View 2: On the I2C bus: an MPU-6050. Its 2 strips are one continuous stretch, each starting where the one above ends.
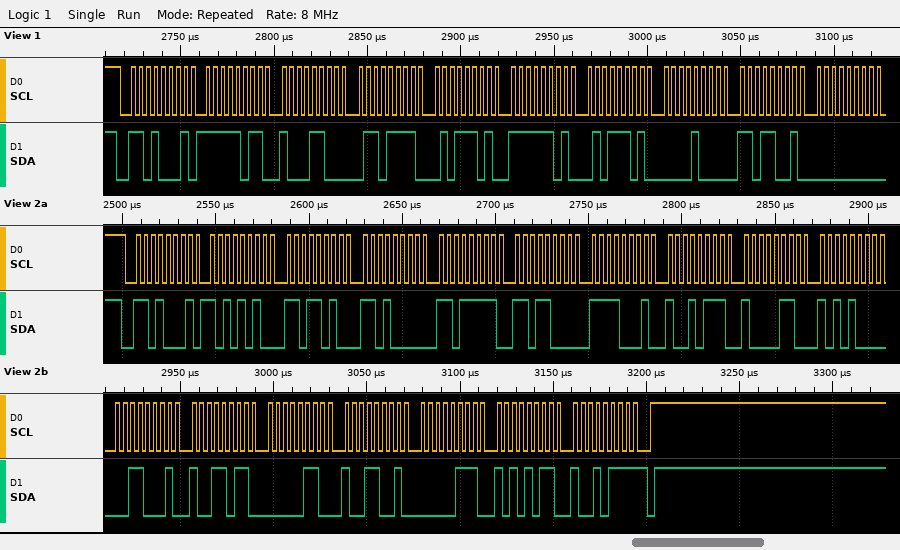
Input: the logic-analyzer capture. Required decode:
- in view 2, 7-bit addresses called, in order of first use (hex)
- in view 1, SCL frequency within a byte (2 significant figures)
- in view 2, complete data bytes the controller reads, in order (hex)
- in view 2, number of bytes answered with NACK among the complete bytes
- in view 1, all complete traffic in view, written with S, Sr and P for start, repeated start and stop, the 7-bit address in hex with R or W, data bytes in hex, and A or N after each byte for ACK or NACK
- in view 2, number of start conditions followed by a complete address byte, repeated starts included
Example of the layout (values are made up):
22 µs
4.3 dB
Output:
0x68
250 kHz
AA DA D0 DF D8 F1 97 86 A8 31 9B 06 99 07 AB 97
1
S 68R A FB A 8C A 6F A 5D A FD A 5D A 08 A D9 A 00 A
1
